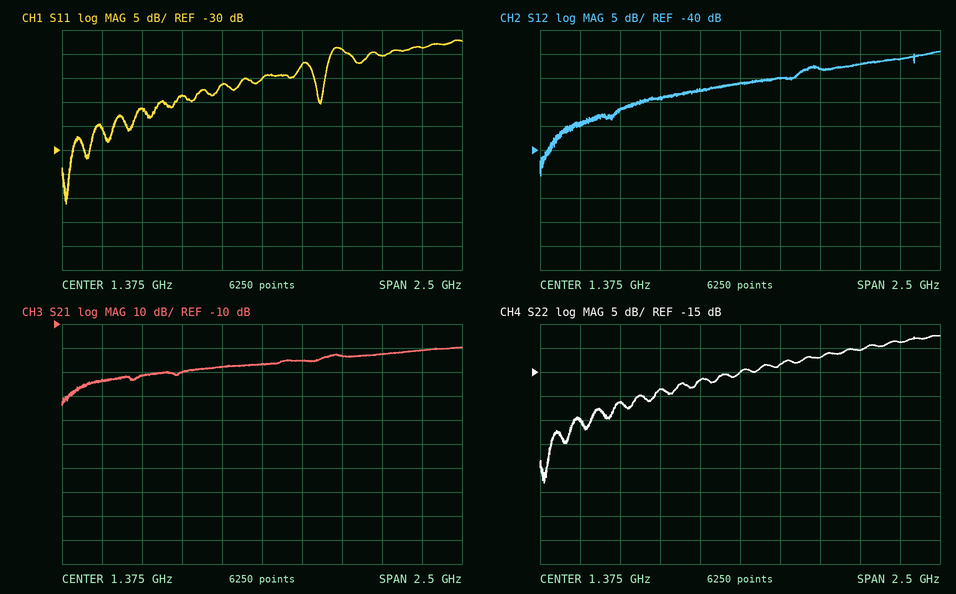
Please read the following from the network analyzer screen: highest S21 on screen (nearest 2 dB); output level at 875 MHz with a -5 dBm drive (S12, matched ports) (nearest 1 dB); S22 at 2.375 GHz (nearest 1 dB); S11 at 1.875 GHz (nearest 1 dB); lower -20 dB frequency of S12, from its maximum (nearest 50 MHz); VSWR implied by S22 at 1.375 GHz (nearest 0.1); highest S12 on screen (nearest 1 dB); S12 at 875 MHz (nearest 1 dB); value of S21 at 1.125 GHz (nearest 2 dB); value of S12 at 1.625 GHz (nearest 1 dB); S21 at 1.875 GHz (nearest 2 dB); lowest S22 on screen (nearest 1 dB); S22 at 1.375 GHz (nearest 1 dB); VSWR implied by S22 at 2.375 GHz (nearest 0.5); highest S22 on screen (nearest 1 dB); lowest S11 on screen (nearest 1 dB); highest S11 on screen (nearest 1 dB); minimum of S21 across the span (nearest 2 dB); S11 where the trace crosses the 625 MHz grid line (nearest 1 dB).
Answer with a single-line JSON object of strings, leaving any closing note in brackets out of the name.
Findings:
{"highest S21 on screen": "-20 dB", "output level at 875 MHz with a -5 dBm drive (S12, matched ports)": "-34 dBm", "S22 at 2.375 GHz": "-9 dB", "S11 at 1.875 GHz": "-9 dB", "lower -20 dB frequency of S12, from its maximum": "200 MHz", "VSWR implied by S22 at 1.375 GHz": "1.4", "highest S12 on screen": "-19 dB", "S12 at 875 MHz": "-29 dB", "value of S21 at 1.125 GHz": "-28 dB", "value of S12 at 1.625 GHz": "-25 dB", "S21 at 1.875 GHz": "-24 dB", "lowest S22 on screen": "-38 dB", "S22 at 1.375 GHz": "-15 dB", "VSWR implied by S22 at 2.375 GHz": "2.0", "highest S22 on screen": "-7 dB", "lowest S11 on screen": "-41 dB", "highest S11 on screen": "-7 dB", "minimum of S21 across the span": "-44 dB", "S11 where the trace crosses the 625 MHz grid line": "-21 dB"}
